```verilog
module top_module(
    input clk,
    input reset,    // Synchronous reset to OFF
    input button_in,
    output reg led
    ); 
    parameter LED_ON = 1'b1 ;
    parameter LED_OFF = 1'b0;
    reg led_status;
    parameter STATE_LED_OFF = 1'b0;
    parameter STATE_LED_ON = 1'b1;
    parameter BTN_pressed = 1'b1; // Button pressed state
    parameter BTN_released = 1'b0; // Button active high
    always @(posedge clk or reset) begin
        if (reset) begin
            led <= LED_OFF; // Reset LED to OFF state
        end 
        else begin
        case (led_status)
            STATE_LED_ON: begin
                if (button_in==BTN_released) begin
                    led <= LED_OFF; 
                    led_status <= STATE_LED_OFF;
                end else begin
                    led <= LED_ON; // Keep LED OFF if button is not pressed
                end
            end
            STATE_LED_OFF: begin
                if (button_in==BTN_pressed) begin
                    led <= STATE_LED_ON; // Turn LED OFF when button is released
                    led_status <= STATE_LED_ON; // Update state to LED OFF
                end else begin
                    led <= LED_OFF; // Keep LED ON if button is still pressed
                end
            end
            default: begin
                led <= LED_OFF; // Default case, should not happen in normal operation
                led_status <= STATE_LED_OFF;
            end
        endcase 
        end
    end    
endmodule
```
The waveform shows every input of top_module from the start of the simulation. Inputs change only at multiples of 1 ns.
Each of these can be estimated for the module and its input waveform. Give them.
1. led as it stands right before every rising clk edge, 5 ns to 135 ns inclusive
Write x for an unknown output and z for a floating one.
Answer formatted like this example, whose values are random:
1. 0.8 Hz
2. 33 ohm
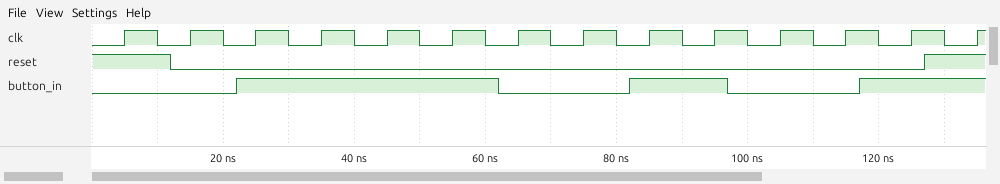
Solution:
1. 0 0 0 1 1 1 1 0 0 1 1 0 0 0
